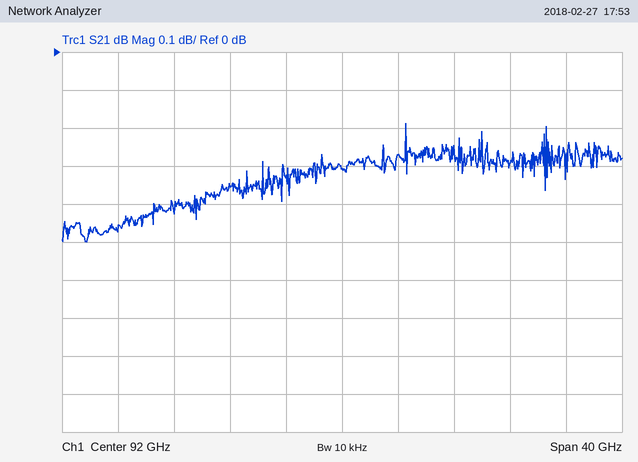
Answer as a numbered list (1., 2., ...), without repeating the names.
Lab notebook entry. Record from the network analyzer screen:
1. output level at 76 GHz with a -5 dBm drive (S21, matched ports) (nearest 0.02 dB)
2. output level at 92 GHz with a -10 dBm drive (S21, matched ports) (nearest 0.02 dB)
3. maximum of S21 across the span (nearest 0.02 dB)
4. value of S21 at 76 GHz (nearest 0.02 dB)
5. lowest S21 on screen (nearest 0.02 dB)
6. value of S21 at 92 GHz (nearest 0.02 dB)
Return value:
1. -5.46 dBm
2. -10.30 dBm
3. -0.18 dB
4. -0.46 dB
5. -0.50 dB
6. -0.30 dB
